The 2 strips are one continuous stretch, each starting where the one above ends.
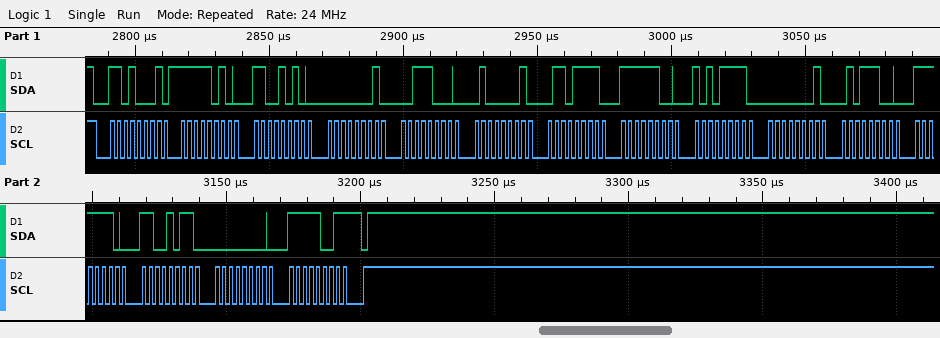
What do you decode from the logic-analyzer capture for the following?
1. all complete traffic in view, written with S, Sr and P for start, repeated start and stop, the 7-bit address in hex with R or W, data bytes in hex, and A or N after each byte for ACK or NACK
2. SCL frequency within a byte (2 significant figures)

S 68R A FA A CA A 01 A 38 A 41 A 6F A FC A AF A 01 A 5C A FE A CB A 00 A F9 N P
400 kHz
